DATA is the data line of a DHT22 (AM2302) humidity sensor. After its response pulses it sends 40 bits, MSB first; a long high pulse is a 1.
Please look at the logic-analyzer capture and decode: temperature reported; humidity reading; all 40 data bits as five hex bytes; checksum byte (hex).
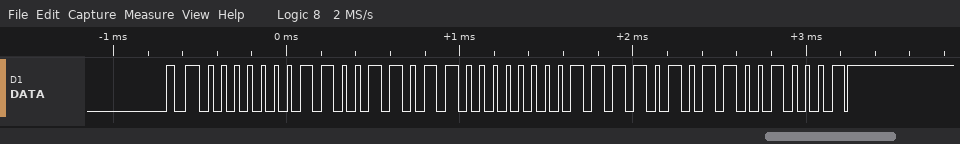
24.5 °C
41.1 %
01 9B 00 F5 91
0x91
